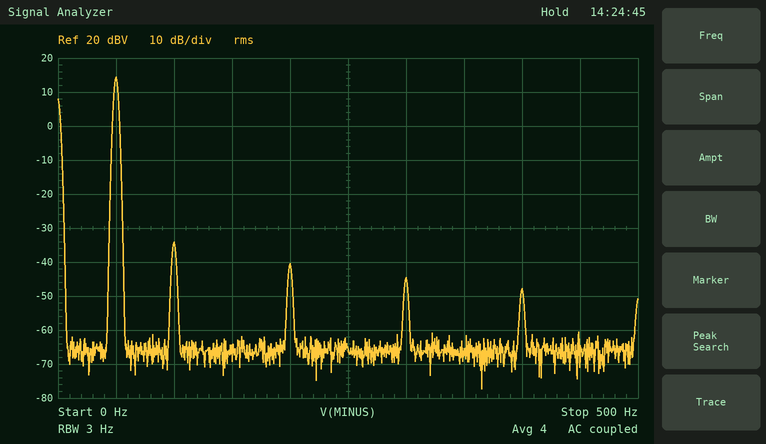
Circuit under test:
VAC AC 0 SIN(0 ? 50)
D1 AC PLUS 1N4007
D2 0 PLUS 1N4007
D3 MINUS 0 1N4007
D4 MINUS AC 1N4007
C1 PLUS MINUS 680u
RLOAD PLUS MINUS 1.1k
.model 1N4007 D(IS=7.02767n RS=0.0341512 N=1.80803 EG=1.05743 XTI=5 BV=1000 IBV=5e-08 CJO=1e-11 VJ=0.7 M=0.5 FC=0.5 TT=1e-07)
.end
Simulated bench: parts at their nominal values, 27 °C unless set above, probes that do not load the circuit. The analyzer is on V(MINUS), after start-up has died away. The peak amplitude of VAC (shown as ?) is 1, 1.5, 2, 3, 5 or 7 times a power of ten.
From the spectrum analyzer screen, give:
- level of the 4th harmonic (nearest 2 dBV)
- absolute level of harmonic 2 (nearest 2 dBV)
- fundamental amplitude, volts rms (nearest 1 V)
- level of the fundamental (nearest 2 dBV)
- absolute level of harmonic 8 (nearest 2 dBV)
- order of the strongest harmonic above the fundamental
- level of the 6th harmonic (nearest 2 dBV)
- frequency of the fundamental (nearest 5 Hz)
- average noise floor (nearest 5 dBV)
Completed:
-40 dBV
-34 dBV
5 V
14 dBV
-48 dBV
2
-44 dBV
50 Hz
-65 dBV
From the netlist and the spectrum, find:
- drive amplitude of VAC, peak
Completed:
15 V
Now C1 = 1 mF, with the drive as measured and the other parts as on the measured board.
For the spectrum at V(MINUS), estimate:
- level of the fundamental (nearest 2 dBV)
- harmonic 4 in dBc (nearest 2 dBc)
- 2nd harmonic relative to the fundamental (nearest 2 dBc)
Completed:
14 dBV
-58 dBc
-52 dBc
